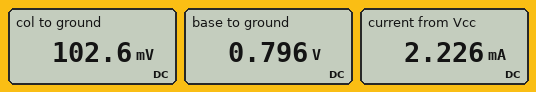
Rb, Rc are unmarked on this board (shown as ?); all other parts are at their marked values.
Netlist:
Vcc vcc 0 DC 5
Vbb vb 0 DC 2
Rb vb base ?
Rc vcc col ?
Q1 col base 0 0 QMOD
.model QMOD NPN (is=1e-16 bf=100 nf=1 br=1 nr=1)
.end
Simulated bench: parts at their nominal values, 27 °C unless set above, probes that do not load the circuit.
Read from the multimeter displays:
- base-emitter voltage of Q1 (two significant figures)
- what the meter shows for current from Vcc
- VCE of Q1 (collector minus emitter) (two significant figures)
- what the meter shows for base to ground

800 mV
2.226 mA
100 mV
0.796 V
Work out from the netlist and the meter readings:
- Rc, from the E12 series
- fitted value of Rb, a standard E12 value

2.2 kΩ
18 kΩ
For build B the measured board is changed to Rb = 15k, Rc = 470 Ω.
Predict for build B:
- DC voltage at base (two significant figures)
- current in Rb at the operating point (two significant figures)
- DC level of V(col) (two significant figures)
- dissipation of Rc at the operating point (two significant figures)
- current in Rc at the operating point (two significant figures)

830 mV
78 µA
1.3 V
29 mW
7.8 mA
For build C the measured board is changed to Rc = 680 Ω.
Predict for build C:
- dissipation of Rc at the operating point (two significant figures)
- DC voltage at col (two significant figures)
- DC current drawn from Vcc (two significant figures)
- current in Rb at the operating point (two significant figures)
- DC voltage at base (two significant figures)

29 mW
550 mV
6.5 mA
65 µA
820 mV
